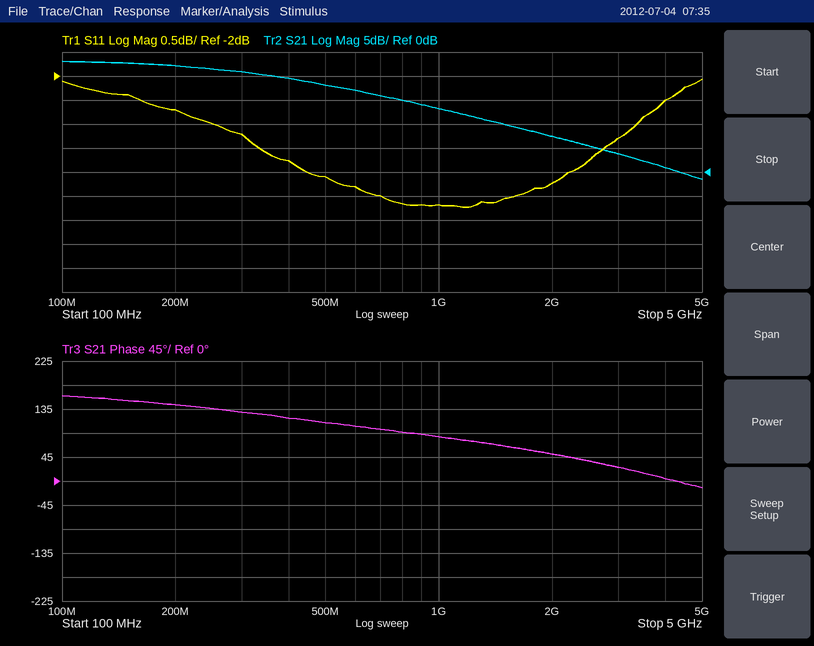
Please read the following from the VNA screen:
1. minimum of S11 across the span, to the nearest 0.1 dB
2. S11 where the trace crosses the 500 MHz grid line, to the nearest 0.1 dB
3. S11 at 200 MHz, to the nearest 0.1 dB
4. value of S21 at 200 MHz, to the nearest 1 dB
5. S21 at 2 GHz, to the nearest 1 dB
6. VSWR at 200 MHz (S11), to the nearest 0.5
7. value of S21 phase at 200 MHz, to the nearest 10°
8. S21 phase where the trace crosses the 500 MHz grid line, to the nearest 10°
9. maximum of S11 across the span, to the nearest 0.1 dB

-4.7 dB
-4.1 dB
-2.7 dB
22 dB
7 dB
6.5
140°
110°
-2.1 dB
